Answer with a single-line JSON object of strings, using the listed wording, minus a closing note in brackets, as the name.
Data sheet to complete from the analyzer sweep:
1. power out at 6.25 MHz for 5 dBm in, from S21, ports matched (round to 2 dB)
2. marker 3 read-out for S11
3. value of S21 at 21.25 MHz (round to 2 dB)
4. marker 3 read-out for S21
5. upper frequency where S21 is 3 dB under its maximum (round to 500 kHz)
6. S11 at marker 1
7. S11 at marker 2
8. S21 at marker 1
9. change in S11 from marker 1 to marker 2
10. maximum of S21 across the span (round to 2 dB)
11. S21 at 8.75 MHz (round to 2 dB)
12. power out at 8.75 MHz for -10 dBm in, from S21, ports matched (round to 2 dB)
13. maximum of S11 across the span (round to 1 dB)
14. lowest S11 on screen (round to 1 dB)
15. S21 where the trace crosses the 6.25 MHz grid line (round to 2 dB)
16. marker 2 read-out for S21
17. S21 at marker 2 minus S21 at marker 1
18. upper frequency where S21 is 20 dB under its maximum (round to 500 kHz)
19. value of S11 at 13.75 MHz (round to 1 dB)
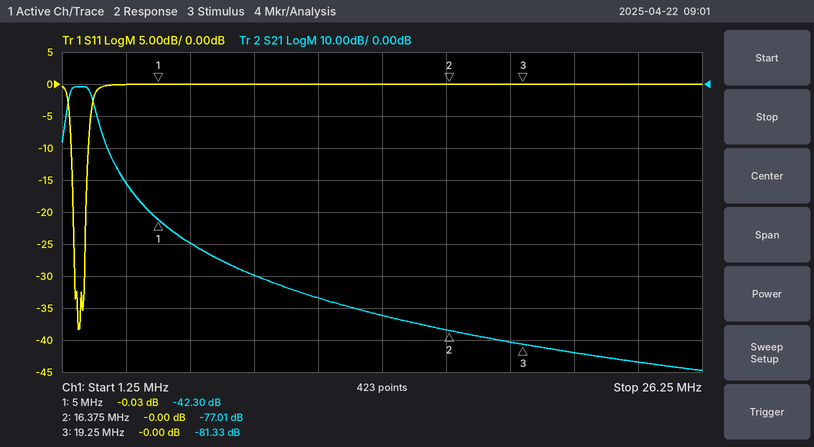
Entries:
{"power out at 6.25 MHz for 5 dBm in, from S21, ports matched": "-44 dBm", "marker 3 read-out for S11": "-0.00 dB", "value of S21 at 21.25 MHz": "-84 dB", "marker 3 read-out for S21": "-81.33 dB", "upper frequency where S21 is 3 dB under its maximum": "2.5 MHz", "S11 at marker 1": "-0.03 dB", "S11 at marker 2": "-0.00 dB", "S21 at marker 1": "-42.30 dB", "change in S11 from marker 1 to marker 2": "0.03 dB", "maximum of S21 across the span": "0 dB", "S21 at 8.75 MHz": "-60 dB", "power out at 8.75 MHz for -10 dBm in, from S21, ports matched": "-70 dBm", "maximum of S11 across the span": "0 dB", "lowest S11 on screen": "-38 dB", "S21 where the trace crosses the 6.25 MHz grid line": "-50 dB", "marker 2 read-out for S21": "-77.01 dB", "S21 at marker 2 minus S21 at marker 1": "-34.71 dB", "upper frequency where S21 is 20 dB under its maximum": "3.0 MHz", "value of S11 at 13.75 MHz": "0 dB"}
